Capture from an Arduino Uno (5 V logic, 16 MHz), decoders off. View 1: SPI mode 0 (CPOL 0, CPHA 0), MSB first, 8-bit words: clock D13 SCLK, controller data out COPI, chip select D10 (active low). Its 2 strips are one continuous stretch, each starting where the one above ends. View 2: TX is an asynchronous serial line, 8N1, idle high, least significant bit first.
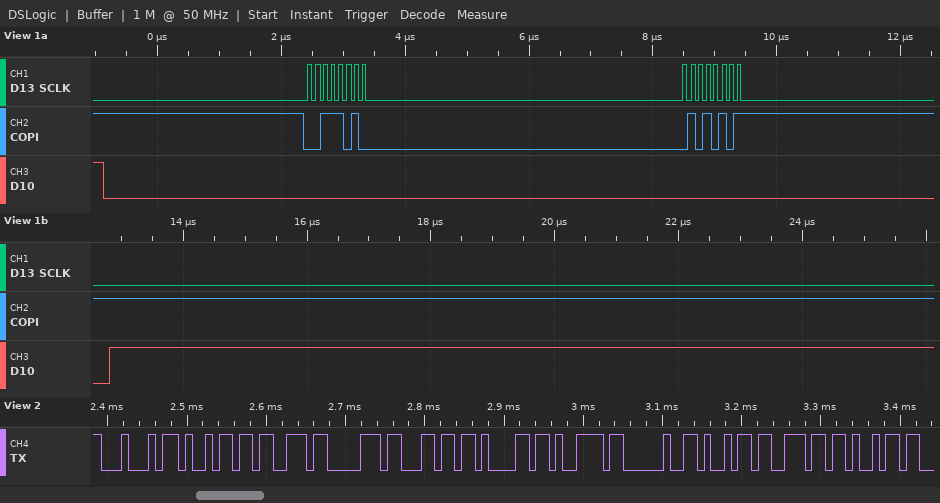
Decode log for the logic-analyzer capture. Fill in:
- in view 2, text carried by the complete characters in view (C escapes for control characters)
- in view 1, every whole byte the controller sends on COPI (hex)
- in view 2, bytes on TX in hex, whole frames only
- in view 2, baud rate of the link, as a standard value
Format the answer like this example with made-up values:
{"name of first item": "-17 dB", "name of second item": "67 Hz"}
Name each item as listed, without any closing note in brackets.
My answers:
{"in view 2, text carried by the complete characters in view": "\"Display ini\"", "in view 1, every whole byte the controller sends on COPI": "0x3A 0x55", "in view 2, bytes on TX in hex, whole frames only": "0x44 0x69 0x73 0x70 0x6C 0x61 0x79 0x20 0x69 0x6E 0x69", "in view 2, baud rate of the link, as a standard value": "115200 baud"}
